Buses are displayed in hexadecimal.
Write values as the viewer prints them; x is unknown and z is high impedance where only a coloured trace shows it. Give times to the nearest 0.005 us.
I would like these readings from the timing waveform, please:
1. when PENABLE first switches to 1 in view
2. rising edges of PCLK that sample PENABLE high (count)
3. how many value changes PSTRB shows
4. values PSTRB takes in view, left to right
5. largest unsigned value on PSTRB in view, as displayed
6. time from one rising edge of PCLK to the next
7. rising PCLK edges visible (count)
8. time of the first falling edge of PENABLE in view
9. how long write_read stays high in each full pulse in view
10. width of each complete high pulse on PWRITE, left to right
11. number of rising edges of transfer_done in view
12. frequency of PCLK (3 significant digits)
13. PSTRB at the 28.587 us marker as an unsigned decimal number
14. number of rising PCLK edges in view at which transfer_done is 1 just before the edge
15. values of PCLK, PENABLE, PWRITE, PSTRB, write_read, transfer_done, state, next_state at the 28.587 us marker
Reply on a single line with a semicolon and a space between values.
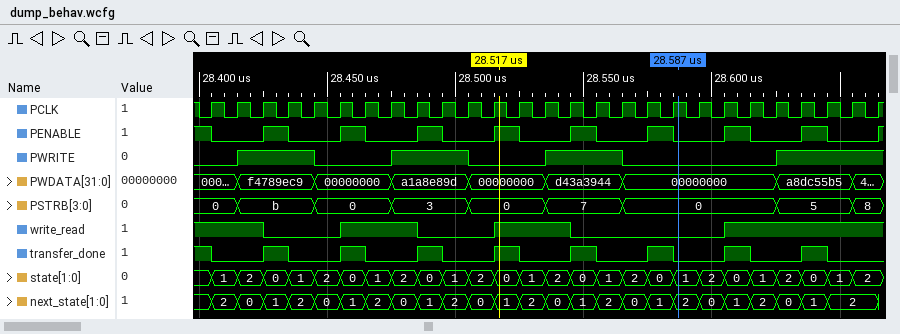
28.425 us; 9; 8; 0, b, 0, 3, 0, 7, 0, 5, 8; b; 0.01 us; 27; 28.405 us; 0.03 us, 0.03 us; 0.03 us, 0.03 us, 0.03 us; 8; 100 MHz; 0; 9; PCLK=1, PENABLE=0, PWRITE=0, PSTRB=0, write_read=0, transfer_done=0, state=1, next_state=2
